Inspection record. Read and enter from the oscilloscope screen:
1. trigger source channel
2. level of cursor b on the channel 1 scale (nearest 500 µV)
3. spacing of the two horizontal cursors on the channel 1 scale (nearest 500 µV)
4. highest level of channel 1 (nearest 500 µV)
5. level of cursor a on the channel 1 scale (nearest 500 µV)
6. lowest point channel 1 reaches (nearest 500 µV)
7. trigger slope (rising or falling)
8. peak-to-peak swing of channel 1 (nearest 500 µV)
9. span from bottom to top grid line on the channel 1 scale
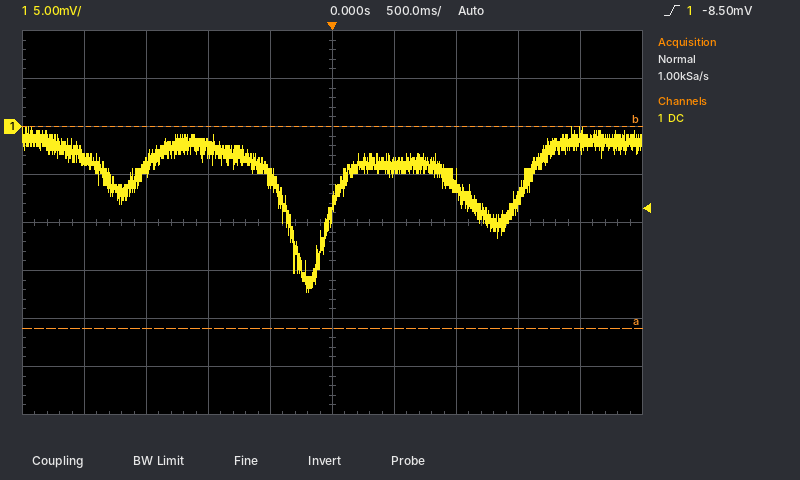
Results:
channel 1
0.0 mV
21.0 mV
0.0 mV
-21.0 mV
-17.0 mV
rising
17.0 mV
40 mV
